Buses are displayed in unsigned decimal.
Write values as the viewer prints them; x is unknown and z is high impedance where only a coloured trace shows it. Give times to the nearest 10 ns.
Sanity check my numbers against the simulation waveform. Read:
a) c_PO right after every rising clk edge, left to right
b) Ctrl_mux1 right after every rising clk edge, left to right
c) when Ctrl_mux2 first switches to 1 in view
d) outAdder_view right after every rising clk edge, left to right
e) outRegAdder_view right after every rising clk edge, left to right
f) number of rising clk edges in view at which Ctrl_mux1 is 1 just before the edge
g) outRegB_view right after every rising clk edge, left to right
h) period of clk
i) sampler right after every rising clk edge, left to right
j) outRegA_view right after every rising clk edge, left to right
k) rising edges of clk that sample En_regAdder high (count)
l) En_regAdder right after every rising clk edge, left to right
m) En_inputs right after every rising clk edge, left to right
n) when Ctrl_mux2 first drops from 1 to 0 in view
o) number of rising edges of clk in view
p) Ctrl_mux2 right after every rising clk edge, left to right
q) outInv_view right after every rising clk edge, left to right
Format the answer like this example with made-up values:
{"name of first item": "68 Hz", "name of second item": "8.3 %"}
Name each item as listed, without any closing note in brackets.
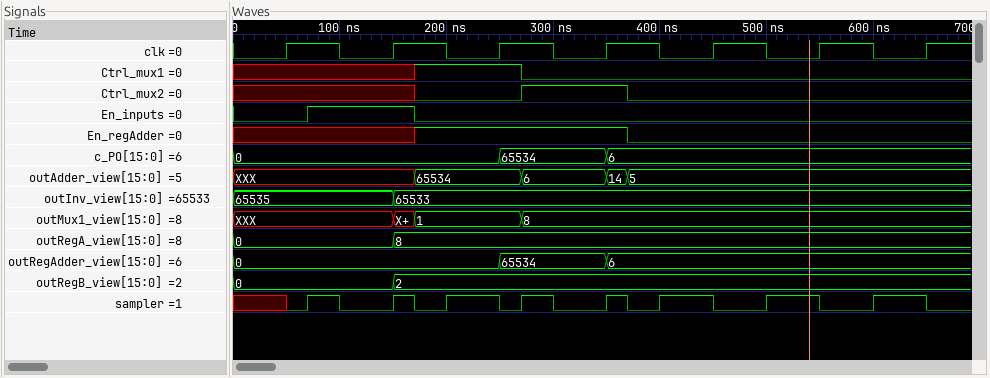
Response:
{"c_PO right after every rising clk edge, left to right": "0, 0, 65534, 6, 6, 6, 6", "Ctrl_mux1 right after every rising clk edge, left to right": "x x 1 0 0 0 0", "when Ctrl_mux2 first switches to 1 in view": "270 ns", "outAdder_view right after every rising clk edge, left to right": "XXX, XXX, 65534, 14, 5, 5, 5", "outRegAdder_view right after every rising clk edge, left to right": "0, 0, 65534, 6, 6, 6, 6", "number of rising clk edges in view at which Ctrl_mux1 is 1 just before the edge": "1", "outRegB_view right after every rising clk edge, left to right": "0, 2, 2, 2, 2, 2, 2", "period of clk": "100 ns", "sampler right after every rising clk edge, left to right": "0 1 0 1 0 0 0", "outRegA_view right after every rising clk edge, left to right": "0, 8, 8, 8, 8, 8, 8", "rising edges of clk that sample En_regAdder high": "2", "En_regAdder right after every rising clk edge, left to right": "x x 1 1 0 0 0", "En_inputs right after every rising clk edge, left to right": "0 1 0 0 0 0 0", "when Ctrl_mux2 first drops from 1 to 0 in view": "370 ns", "number of rising edges of clk in view": "7", "Ctrl_mux2 right after every rising clk edge, left to right": "x x 0 1 0 0 0", "outInv_view right after every rising clk edge, left to right": "65535, 65533, 65533, 65533, 65533, 65533, 65533"}
